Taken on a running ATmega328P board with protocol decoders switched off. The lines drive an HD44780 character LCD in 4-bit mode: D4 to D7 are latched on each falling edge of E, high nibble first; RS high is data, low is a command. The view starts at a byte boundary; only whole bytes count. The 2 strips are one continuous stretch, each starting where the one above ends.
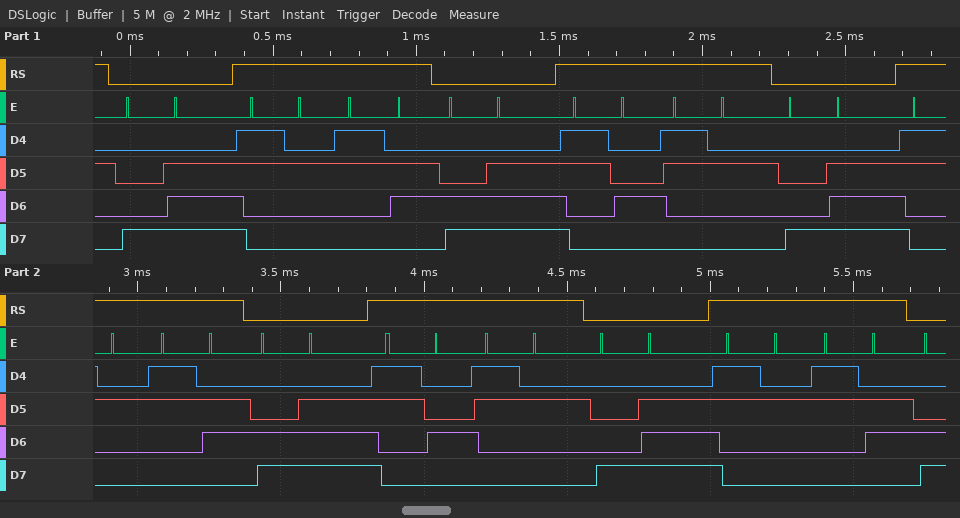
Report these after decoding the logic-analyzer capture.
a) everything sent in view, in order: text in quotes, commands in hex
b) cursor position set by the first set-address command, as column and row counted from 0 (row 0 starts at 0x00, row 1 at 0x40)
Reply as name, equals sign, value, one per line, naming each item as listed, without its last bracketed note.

everything sent in view, in order: text in quotes, commands in hex = 0x8E "26" 0xCE "42" 0x8E "26" 0xCE "42" 0x8E "26"
cursor position set by the first set-address command, as column and row counted from 0 = column 14, row 0
